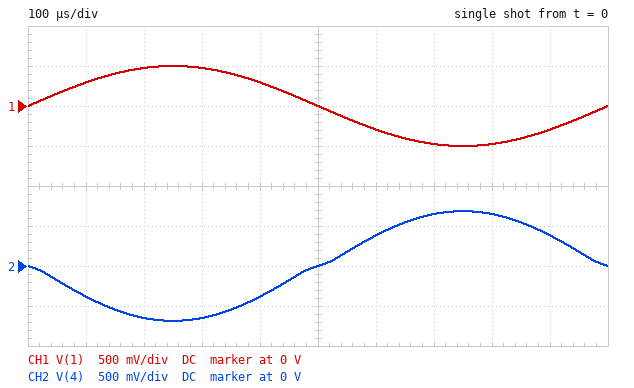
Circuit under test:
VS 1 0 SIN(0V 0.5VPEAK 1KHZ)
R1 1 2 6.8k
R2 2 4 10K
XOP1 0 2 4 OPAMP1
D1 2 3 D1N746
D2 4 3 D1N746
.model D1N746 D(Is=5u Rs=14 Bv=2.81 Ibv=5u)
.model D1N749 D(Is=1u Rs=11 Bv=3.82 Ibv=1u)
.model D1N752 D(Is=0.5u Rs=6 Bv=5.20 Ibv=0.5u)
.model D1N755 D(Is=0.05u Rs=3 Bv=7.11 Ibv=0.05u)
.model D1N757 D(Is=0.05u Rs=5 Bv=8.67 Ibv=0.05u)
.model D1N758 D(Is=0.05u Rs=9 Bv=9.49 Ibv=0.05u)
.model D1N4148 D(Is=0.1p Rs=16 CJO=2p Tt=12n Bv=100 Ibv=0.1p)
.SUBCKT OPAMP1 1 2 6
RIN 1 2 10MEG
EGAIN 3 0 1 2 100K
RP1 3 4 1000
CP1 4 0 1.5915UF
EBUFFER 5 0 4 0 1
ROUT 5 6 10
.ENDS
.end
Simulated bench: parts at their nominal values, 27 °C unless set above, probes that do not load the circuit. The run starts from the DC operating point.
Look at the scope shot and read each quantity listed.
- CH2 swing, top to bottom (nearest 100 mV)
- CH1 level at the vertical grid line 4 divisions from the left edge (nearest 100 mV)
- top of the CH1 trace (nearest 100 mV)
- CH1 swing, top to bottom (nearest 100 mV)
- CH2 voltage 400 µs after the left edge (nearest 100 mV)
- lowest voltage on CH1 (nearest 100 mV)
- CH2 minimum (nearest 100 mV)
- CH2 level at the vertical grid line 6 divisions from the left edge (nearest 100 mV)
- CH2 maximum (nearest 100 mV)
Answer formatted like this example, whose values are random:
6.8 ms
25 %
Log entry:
1.4 V
300 mV
500 mV
1.0 V
-400 mV
-500 mV
-700 mV
400 mV
700 mV
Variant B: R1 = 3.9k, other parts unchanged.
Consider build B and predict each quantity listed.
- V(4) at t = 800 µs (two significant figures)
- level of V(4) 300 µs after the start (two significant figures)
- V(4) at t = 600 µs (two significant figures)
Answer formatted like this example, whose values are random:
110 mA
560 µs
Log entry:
1.2 V
-1.2 V
700 mV
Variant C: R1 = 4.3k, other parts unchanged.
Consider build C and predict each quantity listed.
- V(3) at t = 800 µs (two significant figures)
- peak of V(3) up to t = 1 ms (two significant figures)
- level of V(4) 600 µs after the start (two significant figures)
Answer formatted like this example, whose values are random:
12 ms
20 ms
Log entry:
1.0 V
1.1 V
630 mV
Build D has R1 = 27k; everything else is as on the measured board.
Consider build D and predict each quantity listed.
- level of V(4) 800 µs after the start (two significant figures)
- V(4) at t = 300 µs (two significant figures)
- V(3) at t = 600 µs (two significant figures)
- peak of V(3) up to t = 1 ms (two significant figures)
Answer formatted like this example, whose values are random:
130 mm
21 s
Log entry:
130 mV
-130 mV
50 mV
120 mV
